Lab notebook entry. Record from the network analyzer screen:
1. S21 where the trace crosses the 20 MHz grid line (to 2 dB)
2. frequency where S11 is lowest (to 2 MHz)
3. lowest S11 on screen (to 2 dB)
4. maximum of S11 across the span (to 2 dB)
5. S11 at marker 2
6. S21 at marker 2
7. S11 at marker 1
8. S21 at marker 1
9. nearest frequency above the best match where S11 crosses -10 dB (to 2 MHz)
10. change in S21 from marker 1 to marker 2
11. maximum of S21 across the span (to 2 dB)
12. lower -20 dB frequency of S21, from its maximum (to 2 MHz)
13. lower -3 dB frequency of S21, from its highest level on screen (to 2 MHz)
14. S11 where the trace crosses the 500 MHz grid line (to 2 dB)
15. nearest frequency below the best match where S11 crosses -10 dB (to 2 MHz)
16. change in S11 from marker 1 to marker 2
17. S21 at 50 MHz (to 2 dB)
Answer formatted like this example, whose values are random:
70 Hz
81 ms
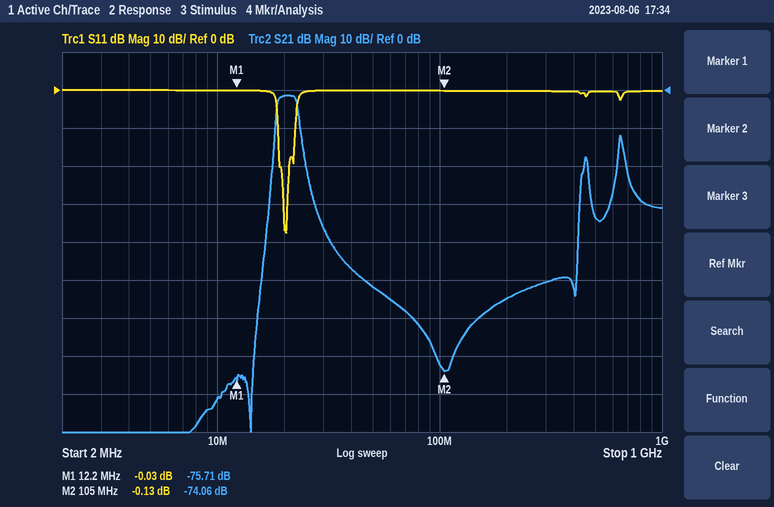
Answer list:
-2 dB
20 MHz
-38 dB
0 dB
-0.13 dB
-74.06 dB
-0.03 dB
-75.71 dB
22 MHz
1.65 dB
-2 dB
18 MHz
18 MHz
0 dB
18 MHz
-0.10 dB
-52 dB
